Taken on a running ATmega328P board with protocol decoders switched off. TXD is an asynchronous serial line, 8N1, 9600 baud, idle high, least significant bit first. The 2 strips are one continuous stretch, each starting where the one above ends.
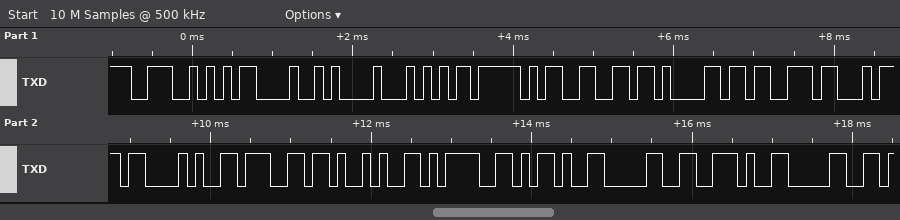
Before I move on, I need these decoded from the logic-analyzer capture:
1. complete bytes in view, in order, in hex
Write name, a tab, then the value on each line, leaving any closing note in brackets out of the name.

complete bytes in view, in order, in hex	0x4E 0x0D 0x0A 0x54 0x5F 0x66 0x61 0x73 0x74 0x28 0x67 0x29 0x3D 0x2D 0x30 0x2E 0x30
